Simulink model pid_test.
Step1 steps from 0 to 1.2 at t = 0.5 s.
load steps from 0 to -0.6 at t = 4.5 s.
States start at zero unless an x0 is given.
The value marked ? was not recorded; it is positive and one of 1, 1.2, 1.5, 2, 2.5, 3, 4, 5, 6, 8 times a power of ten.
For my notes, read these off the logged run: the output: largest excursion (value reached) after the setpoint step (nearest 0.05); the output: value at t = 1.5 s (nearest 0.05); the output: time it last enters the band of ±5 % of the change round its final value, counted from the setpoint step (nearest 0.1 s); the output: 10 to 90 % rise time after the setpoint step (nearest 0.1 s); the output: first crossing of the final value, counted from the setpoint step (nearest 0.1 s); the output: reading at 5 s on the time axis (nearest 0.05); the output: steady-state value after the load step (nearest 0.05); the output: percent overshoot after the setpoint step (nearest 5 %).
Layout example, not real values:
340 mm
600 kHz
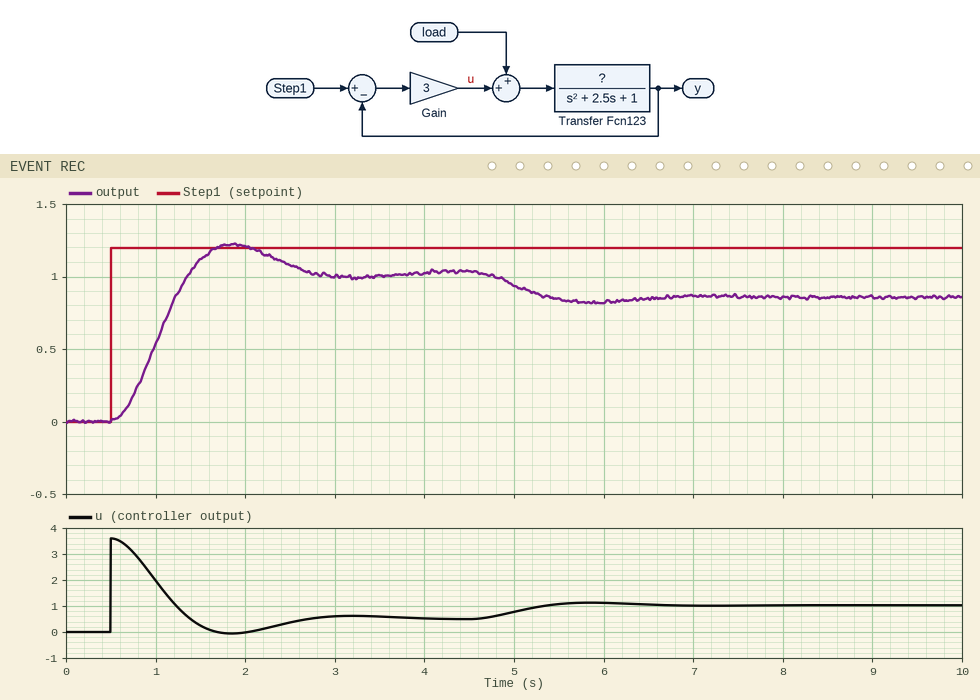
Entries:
1.20
1.10
2.0 s
0.6 s
0.9 s
0.95
0.85
20 %
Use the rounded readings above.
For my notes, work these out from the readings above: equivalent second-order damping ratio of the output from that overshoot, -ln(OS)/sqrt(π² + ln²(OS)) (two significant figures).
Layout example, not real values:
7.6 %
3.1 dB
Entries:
0.46
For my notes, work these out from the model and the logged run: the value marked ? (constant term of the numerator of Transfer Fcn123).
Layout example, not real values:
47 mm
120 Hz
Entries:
2
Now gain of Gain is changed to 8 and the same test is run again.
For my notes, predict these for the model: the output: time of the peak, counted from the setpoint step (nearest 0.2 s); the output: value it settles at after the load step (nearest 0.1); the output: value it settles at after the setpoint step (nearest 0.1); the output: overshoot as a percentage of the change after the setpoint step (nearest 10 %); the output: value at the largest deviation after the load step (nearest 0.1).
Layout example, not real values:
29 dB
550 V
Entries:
0.8 s
1.1
1.1
40 %
1.0
